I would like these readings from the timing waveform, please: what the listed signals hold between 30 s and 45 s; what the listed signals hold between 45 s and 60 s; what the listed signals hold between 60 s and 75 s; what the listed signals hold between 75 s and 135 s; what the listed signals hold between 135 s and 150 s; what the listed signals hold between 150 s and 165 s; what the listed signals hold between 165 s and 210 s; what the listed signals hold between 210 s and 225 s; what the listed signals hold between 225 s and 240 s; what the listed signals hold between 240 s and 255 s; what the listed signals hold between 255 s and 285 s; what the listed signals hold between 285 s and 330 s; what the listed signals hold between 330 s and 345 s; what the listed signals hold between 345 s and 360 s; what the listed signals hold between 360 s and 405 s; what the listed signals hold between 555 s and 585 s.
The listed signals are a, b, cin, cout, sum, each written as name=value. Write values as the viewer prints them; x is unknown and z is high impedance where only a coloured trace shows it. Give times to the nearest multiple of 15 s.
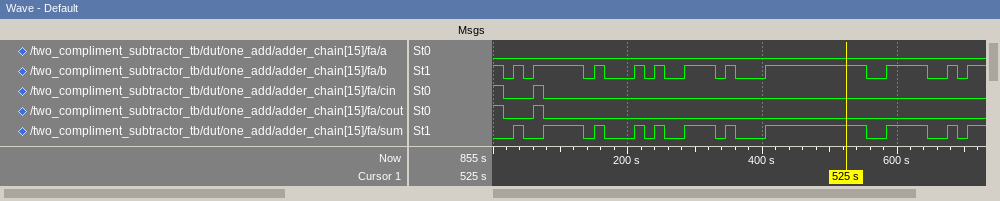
a=0, b=1, cin=0, cout=0, sum=1
a=0, b=0, cin=0, cout=0, sum=0
a=0, b=1, cin=1, cout=1, sum=0
a=0, b=1, cin=0, cout=0, sum=1
a=0, b=0, cin=0, cout=0, sum=0
a=0, b=1, cin=0, cout=0, sum=1
a=0, b=0, cin=0, cout=0, sum=0
a=0, b=1, cin=0, cout=0, sum=1
a=0, b=0, cin=0, cout=0, sum=0
a=0, b=1, cin=0, cout=0, sum=1
a=0, b=0, cin=0, cout=0, sum=0
a=0, b=1, cin=0, cout=0, sum=1
a=0, b=0, cin=0, cout=0, sum=0
a=0, b=1, cin=0, cout=0, sum=1
a=0, b=0, cin=0, cout=0, sum=0
a=0, b=0, cin=0, cout=0, sum=0
